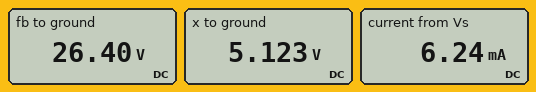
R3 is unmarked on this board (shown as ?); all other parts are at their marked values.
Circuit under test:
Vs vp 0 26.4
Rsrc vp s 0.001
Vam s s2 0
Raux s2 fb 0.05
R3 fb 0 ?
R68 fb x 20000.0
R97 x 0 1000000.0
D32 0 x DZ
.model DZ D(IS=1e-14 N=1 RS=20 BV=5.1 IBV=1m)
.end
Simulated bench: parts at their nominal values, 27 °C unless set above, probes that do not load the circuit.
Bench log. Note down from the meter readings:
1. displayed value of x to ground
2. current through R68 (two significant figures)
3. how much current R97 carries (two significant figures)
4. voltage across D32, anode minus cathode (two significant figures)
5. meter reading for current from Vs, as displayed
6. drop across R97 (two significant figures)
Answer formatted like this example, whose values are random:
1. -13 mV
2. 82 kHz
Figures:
1. 5.123 V
2. 1.1 mA
3. 5.1 µA
4. -5.1 V
5. 6.24 mA
6. 5.1 V
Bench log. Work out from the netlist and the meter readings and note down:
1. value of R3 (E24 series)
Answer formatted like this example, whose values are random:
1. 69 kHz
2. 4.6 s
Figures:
1. 5.1 kΩ
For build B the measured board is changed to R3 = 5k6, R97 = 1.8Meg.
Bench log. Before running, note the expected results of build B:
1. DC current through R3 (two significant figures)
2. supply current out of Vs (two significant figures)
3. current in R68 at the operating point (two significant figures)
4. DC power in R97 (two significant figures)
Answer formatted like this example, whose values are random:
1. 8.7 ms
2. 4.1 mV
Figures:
1. 4.7 mA
2. 5.8 mA
3. 1.1 mA
4. 15 µW
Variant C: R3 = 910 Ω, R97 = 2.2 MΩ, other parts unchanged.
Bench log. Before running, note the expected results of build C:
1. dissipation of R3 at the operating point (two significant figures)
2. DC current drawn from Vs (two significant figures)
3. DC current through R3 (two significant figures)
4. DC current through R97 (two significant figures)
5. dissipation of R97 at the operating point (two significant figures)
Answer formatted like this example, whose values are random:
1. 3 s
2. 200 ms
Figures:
1. 770 mW
2. 30 mA
3. 29 mA
4. 2.3 µA
5. 12 µW
